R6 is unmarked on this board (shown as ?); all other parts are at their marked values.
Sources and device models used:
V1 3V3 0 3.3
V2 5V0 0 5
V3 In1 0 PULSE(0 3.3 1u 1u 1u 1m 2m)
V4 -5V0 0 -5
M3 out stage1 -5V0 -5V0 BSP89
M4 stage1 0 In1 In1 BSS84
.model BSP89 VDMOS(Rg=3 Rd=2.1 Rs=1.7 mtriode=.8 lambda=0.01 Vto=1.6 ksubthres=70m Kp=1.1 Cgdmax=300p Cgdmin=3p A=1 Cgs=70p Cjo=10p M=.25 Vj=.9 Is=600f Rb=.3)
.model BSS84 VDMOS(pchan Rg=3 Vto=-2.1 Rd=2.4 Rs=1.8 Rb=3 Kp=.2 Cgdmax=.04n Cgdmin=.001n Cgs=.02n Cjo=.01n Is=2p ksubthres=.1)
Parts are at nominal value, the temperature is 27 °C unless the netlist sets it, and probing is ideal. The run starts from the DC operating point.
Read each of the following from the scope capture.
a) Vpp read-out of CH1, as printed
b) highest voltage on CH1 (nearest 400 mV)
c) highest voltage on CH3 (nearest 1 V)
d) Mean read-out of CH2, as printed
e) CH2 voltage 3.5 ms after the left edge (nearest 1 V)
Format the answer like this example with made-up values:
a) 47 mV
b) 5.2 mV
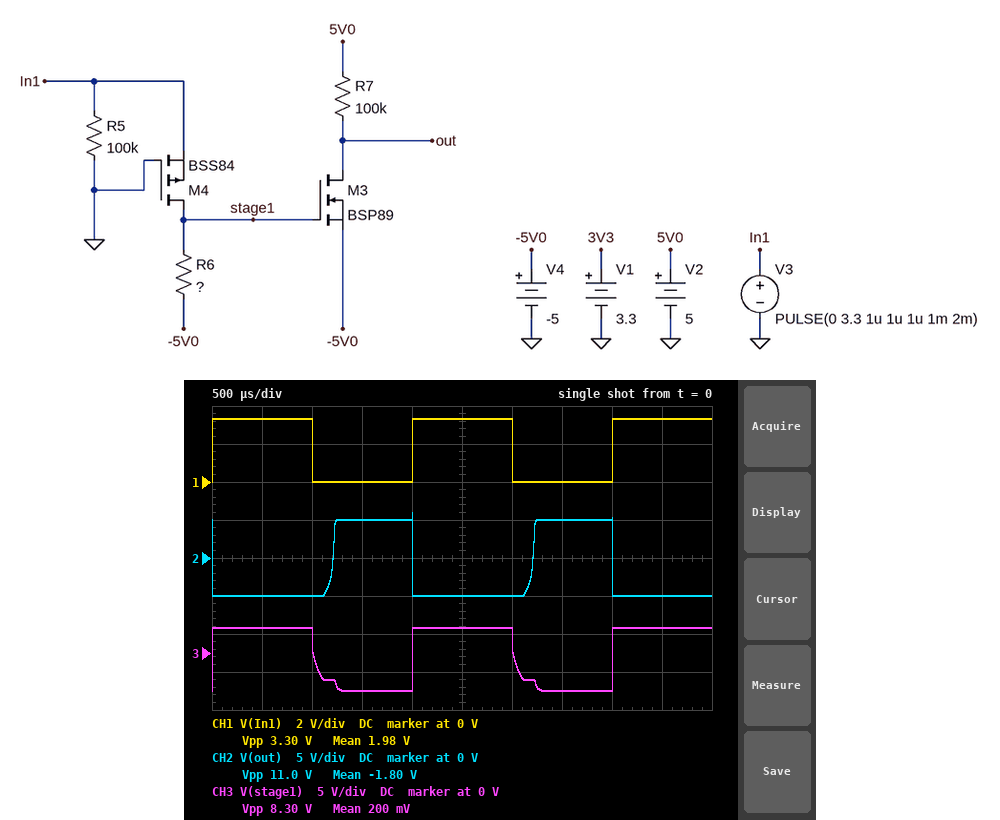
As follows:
a) 3.30 V
b) 3.2 V
c) 3 V
d) -1.80 V
e) 5 V
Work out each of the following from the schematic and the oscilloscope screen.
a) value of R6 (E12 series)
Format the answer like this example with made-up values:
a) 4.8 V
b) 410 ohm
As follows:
a) 220 kΩ
